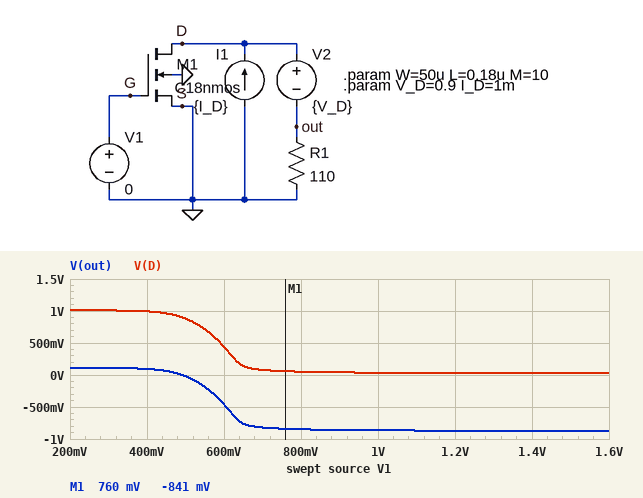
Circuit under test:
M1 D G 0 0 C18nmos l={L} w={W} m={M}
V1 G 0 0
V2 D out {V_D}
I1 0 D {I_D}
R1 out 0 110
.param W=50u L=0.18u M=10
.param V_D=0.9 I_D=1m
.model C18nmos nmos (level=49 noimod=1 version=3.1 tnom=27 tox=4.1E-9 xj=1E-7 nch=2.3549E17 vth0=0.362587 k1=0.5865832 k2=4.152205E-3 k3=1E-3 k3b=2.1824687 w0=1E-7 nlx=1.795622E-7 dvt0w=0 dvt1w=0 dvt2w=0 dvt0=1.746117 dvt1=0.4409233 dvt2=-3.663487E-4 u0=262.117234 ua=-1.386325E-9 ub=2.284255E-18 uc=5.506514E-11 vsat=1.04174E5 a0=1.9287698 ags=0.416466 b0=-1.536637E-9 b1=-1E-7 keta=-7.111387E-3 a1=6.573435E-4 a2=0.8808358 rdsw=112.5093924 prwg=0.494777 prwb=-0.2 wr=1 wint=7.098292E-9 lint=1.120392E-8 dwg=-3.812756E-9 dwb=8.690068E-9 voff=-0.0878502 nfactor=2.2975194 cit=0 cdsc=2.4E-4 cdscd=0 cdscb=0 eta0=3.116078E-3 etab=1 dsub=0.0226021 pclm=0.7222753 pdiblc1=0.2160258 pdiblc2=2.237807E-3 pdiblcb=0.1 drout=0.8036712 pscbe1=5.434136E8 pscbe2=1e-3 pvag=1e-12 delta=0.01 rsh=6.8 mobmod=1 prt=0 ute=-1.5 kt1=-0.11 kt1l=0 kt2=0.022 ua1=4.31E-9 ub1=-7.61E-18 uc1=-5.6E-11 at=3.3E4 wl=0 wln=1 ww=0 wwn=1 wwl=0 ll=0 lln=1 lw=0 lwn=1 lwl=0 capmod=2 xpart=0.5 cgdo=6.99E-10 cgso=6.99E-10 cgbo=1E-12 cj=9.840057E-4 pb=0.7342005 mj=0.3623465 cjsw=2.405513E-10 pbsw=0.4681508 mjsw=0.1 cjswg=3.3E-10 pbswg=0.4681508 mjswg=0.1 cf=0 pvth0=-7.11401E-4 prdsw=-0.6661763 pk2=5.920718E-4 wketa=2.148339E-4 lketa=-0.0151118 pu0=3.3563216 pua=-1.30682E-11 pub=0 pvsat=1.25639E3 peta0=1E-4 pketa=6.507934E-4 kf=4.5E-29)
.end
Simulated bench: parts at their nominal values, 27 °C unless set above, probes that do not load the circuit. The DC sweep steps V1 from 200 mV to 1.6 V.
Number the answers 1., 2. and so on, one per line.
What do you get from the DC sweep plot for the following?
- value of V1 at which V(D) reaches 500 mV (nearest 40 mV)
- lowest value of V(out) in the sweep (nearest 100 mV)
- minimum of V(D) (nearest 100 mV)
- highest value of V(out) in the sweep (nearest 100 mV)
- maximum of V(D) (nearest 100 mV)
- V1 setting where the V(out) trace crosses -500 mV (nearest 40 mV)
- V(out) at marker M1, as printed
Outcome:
1. 600 mV
2. -900 mV
3. 0 V
4. 100 mV
5. 1.0 V
6. 600 mV
7. -841 mV
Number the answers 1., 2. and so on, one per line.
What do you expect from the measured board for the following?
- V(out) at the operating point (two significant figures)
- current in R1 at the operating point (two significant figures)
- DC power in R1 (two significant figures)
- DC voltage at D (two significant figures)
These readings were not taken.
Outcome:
1. 110 mV
2. 1.0 mA
3. 110 µW
4. 1.0 V
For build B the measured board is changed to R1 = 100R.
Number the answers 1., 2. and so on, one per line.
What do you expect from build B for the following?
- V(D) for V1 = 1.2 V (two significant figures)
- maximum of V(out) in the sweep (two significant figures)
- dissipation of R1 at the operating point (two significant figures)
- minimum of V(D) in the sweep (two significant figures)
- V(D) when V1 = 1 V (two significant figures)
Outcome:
1. 33 mV
2. 100 mV
3. 100 µW
4. 28 mV
5. 39 mV
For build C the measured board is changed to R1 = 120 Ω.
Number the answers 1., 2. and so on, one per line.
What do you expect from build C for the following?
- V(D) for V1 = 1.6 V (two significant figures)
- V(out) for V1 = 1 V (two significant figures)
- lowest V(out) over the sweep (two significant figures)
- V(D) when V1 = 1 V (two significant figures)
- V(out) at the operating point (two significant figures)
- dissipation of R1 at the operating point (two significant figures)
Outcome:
1. 24 mV
2. -870 mV
3. -880 mV
4. 33 mV
5. 120 mV
6. 120 µW
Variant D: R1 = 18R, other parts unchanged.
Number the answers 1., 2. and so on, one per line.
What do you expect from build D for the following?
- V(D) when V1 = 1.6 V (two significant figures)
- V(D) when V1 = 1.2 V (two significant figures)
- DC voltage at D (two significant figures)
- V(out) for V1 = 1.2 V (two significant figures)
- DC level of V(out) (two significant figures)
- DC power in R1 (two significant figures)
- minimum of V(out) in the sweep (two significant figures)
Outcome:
1. 130 mV
2. 160 mV
3. 920 mV
4. -740 mV
5. 18 mV
6. 18 µW
7. -770 mV
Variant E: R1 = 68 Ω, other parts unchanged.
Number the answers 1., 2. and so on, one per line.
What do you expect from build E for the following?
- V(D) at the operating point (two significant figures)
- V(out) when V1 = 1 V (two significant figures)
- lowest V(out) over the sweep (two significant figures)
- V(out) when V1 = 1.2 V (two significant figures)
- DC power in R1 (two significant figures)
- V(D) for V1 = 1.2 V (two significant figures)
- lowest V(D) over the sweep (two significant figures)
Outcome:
1. 970 mV
2. -840 mV
3. -860 mV
4. -850 mV
5. 68 µW
6. 47 mV
7. 40 mV
